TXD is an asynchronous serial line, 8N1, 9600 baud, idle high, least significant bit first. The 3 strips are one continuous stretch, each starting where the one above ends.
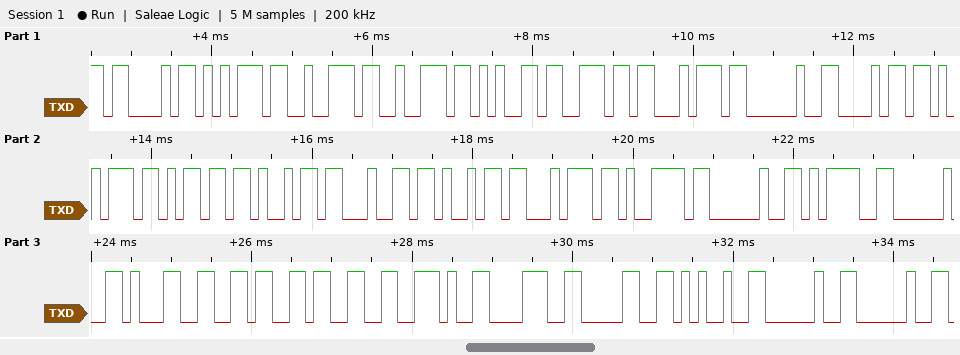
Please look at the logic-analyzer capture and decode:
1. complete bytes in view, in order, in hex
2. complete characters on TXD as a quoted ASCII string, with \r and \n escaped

0x43 0x75 0x72 0x72 0x65 0x6E 0x74 0x20 0x68 0x75 0x6D 0x69 0x64 0x69 0x74 0x79 0x20 0x3D 0x20 0x31 0x36 0x33 0x2E 0x38 0x30 0x25 0x20 0x20
"Current humidity = 163.80%  "
